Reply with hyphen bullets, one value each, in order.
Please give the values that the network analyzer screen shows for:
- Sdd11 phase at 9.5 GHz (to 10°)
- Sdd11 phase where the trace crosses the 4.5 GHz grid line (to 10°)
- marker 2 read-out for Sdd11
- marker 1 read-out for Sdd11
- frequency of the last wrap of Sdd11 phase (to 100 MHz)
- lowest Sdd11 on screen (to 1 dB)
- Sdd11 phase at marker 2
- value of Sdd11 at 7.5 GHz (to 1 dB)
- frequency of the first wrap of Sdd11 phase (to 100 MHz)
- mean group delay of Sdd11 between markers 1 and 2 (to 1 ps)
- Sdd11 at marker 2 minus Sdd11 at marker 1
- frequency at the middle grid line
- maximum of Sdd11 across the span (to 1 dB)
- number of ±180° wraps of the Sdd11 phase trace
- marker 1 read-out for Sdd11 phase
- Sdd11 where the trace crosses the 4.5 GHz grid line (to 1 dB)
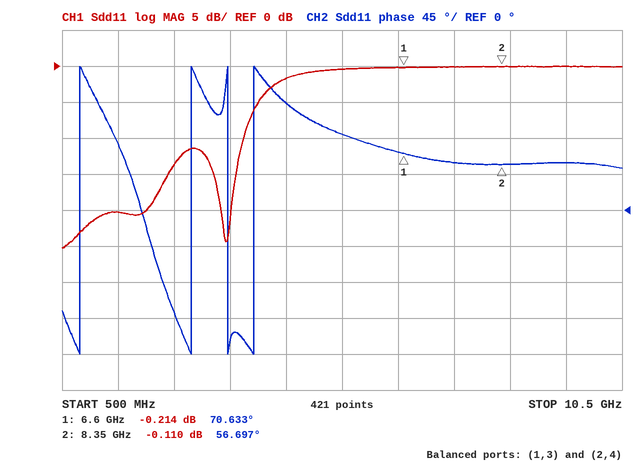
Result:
- 60°
- 130°
- -0.110 dB
- -0.214 dB
- 3.9 GHz
- -25 dB
- 56.697°
- 0 dB
- 800 MHz
- 22 ps
- 0.104 dB
- 5.5 GHz
- 0 dB
- 4
- 70.633°
- -2 dB
